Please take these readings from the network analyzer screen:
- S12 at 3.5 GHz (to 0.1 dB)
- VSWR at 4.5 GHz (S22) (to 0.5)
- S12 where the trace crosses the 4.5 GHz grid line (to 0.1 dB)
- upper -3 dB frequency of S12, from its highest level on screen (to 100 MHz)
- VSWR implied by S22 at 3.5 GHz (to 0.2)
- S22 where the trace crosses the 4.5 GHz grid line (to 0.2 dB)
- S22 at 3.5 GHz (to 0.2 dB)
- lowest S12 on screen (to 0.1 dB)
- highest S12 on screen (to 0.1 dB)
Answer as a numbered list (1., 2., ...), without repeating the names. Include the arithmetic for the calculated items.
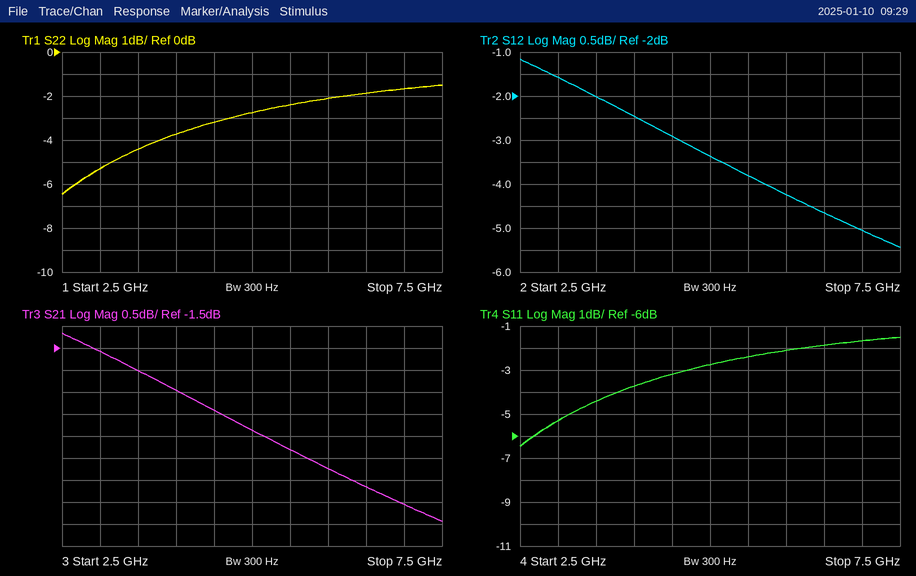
1. -2.0 dB
2. |Γ| = 10^(-3.2/20) = 0.6918; VSWR = (1 + 0.6918)/(1 − 0.6918) ≈ 5.5
3. -2.9 dB
4. 5.9 GHz
5. |Γ| = 10^(-4.4/20) = 0.6026; VSWR = (1 + 0.6026)/(1 − 0.6026) ≈ 4.0
6. -3.2 dB
7. -4.4 dB
8. -5.4 dB
9. -1.2 dB
